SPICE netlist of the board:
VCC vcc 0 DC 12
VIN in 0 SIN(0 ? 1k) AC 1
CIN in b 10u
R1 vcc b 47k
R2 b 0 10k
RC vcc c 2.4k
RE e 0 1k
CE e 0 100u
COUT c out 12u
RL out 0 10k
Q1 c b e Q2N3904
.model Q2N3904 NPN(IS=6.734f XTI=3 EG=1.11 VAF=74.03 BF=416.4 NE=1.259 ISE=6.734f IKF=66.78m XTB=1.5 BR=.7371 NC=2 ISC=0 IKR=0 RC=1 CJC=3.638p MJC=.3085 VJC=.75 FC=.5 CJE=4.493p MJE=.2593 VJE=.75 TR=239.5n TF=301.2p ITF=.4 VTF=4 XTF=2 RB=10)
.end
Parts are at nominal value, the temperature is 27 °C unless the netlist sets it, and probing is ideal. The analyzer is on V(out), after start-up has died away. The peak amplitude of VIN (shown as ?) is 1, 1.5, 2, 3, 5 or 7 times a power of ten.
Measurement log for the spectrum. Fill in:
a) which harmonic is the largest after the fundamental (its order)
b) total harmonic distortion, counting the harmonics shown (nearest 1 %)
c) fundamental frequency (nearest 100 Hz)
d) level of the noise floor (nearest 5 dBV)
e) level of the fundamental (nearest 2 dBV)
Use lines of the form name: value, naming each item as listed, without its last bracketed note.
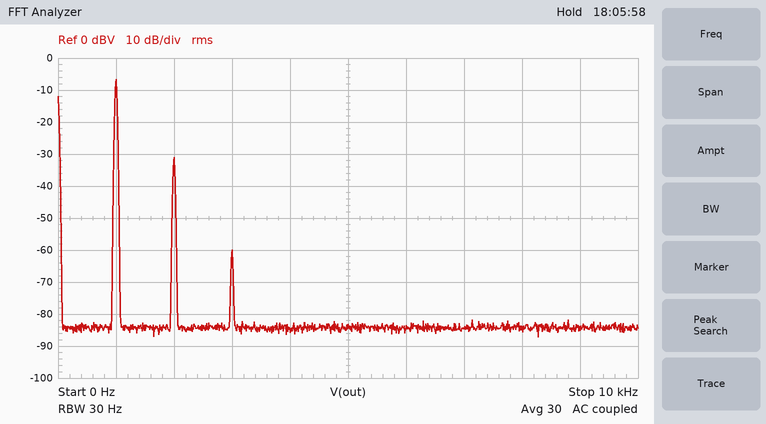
which harmonic is the largest after the fundamental: 2
total harmonic distortion, counting the harmonics shown: 6 %
fundamental frequency: 1.0 kHz
level of the noise floor: -85 dBV
level of the fundamental: -6 dBV
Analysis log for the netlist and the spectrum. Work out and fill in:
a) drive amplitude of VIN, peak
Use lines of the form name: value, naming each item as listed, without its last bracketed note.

drive amplitude of VIN, peak: 7 mV
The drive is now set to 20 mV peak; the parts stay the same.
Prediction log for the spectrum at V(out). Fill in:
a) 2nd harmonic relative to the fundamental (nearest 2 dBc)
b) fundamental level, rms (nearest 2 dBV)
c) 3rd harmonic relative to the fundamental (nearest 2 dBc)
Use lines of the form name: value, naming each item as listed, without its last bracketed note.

2nd harmonic relative to the fundamental: -16 dBc
fundamental level, rms: 2 dBV
3rd harmonic relative to the fundamental: -36 dBc
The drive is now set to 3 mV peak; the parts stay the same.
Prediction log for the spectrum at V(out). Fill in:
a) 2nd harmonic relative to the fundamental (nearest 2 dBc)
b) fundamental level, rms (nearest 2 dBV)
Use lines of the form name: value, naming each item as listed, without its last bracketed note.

2nd harmonic relative to the fundamental: -32 dBc
fundamental level, rms: -14 dBV
